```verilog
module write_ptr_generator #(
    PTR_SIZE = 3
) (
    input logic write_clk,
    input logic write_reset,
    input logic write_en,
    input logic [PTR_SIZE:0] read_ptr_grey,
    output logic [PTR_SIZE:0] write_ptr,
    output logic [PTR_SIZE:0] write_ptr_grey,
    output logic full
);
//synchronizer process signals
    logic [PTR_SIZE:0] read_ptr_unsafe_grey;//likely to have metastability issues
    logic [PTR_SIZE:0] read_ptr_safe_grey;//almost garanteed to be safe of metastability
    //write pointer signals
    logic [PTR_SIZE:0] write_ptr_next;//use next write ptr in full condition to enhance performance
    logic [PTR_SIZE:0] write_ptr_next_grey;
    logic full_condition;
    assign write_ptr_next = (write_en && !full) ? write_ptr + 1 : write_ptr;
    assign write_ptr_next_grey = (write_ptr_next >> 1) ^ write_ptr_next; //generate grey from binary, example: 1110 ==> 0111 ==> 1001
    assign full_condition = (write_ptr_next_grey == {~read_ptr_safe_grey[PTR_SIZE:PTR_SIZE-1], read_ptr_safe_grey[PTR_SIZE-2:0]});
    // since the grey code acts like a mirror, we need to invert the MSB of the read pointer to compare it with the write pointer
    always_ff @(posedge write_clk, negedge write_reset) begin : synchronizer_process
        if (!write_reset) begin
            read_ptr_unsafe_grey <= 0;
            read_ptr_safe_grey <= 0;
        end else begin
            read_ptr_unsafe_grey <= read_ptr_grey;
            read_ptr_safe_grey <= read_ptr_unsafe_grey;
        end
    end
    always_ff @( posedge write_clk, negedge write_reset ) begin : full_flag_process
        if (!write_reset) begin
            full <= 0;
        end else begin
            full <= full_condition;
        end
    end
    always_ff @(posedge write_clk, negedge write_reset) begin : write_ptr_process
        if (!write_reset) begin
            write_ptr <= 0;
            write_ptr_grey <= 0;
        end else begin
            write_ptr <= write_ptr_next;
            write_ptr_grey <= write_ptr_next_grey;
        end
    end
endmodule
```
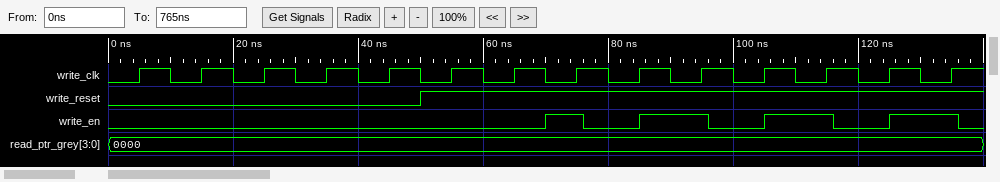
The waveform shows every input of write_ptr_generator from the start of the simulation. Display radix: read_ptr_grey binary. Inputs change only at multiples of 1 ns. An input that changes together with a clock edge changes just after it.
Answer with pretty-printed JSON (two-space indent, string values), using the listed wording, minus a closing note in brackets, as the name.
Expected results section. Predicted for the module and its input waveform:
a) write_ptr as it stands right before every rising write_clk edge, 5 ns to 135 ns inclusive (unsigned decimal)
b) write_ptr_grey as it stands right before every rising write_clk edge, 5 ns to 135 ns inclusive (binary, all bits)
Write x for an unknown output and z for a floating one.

{
  "write_ptr as it stands right before every rising write_clk edge, 5 ns to 135 ns inclusive": "0, 0, 0, 0, 0, 0, 0, 0, 1, 1, 2, 2, 3, 3",
  "write_ptr_grey as it stands right before every rising write_clk edge, 5 ns to 135 ns inclusive": "0000, 0000, 0000, 0000, 0000, 0000, 0000, 0000, 0001, 0001, 0011, 0011, 0010, 0010"
}
